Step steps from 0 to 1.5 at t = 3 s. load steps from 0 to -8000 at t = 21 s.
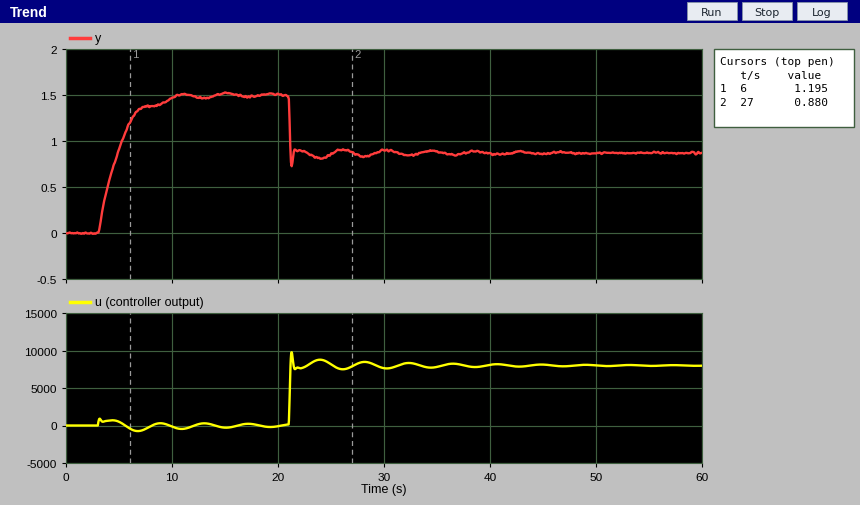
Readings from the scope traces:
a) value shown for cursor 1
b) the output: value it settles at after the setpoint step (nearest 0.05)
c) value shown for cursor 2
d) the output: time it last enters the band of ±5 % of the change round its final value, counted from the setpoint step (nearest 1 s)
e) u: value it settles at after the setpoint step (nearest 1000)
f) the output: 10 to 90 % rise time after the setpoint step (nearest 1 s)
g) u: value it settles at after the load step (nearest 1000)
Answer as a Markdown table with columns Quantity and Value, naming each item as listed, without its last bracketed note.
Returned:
| Quantity | Value |
|---|---|
| value shown for cursor 1 | 1.195 |
| the output: value it settles at after the setpoint step | 1.50 |
| value shown for cursor 2 | 0.880 |
| the output: time it last enters the band of ±5 % of the change round its final value, counted from the setpoint step | 6 s |
| u: value it settles at after the setpoint step | 0 |
| the output: 10 to 90 % rise time after the setpoint step | 4 s |
| u: value it settles at after the load step | 8000 |
